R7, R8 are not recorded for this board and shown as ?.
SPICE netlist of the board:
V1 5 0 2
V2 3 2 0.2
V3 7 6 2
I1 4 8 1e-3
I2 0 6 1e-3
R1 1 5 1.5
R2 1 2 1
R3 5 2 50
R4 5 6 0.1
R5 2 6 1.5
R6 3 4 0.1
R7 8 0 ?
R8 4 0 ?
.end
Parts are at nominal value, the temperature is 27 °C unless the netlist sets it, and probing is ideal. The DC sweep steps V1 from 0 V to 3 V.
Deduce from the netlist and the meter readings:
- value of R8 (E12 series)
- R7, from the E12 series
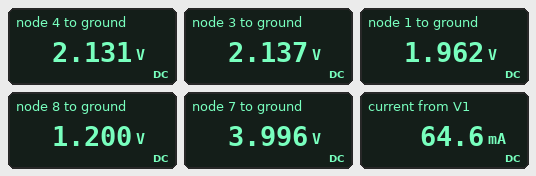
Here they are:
33 Ω
1.2 kΩ
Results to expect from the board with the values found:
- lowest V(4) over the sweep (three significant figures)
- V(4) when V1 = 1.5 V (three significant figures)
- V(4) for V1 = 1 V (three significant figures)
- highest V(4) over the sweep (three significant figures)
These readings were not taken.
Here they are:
193 mV
1.65 V
1.16 V
3.10 V
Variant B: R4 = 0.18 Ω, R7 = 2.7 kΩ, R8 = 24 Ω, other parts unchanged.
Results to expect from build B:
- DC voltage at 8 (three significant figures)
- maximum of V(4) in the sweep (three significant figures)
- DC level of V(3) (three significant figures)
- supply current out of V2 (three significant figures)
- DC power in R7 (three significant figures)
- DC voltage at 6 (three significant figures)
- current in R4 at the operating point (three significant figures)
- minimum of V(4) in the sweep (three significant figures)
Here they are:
2.70 V
3.06 V
2.11 V
88.7 mA
2.70 mW
1.99 V
51.0 mA
190 mV
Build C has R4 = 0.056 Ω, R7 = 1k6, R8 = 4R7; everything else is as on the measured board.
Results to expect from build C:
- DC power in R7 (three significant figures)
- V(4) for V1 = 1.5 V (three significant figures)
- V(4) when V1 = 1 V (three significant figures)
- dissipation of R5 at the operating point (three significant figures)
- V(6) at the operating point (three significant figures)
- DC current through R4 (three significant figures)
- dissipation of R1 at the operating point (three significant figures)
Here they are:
1.60 mW
1.39 V
982 mV
80.9 mW
1.99 V
231 mA
31.3 mW
